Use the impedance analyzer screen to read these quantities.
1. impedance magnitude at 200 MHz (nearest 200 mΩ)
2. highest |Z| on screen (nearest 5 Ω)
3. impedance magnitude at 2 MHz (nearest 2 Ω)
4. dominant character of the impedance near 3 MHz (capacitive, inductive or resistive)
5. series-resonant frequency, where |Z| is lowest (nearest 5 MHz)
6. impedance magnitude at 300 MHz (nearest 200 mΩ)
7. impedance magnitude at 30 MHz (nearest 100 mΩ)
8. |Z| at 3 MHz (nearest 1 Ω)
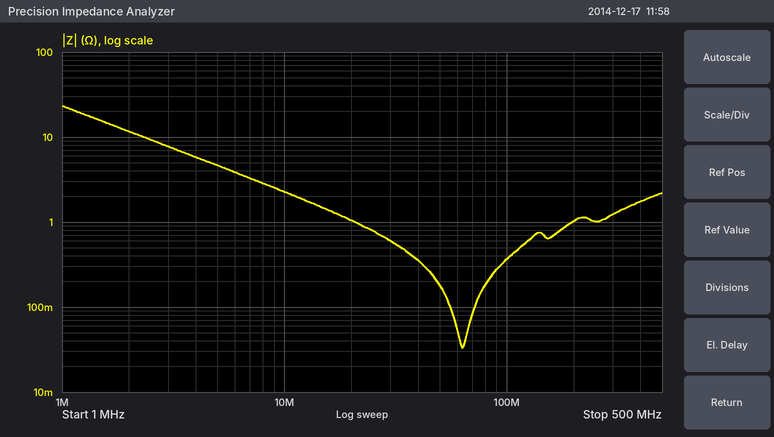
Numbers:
1.0 Ω
25 Ω
12 Ω
capacitive
65 MHz
1.2 Ω
600 mΩ
8 Ω
